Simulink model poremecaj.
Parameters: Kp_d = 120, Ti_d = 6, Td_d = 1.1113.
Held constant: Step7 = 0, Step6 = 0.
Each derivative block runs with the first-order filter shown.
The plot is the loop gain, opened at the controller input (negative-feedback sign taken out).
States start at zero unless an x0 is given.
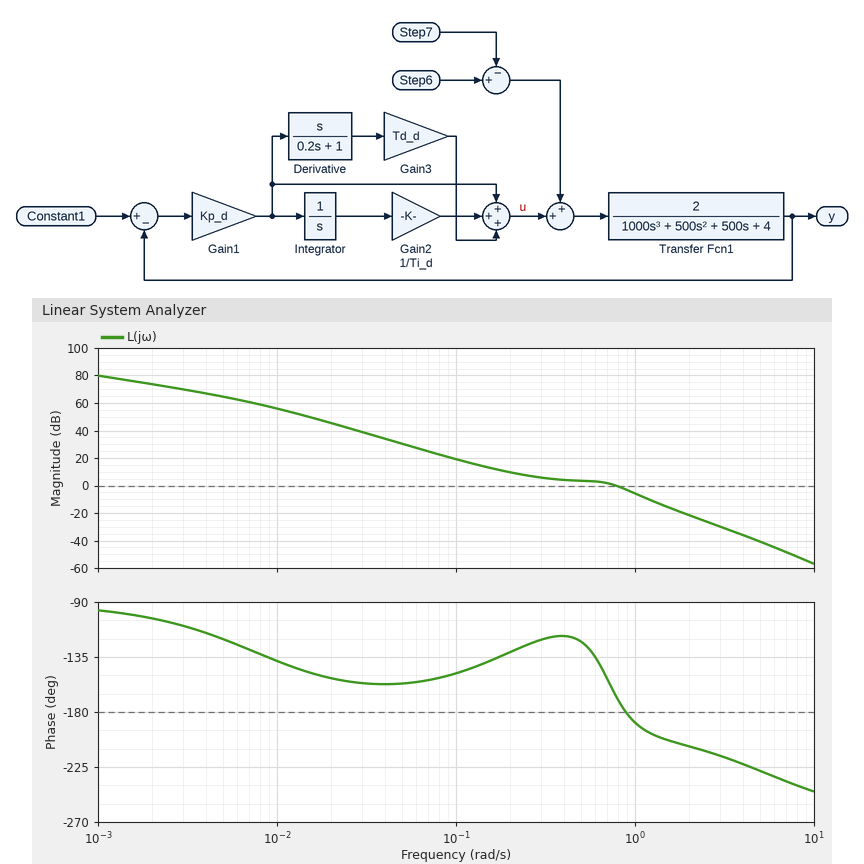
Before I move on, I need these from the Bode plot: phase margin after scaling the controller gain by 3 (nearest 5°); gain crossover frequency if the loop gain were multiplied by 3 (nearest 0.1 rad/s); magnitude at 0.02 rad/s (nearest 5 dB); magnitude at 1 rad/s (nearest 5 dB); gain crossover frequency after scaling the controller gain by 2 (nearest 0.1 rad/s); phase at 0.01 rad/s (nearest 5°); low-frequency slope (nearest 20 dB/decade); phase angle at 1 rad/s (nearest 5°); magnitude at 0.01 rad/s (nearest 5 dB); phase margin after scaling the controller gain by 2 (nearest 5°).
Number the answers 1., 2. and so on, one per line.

1. -15°
2. 1.2 rad/s
3. 45 dB
4. -5 dB
5. 1.0 rad/s
6. -140°
7. -20 dB/decade
8. -190°
9. 55 dB
10. -10°
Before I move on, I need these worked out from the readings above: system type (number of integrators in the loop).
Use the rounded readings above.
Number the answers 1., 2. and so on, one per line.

1. 1
